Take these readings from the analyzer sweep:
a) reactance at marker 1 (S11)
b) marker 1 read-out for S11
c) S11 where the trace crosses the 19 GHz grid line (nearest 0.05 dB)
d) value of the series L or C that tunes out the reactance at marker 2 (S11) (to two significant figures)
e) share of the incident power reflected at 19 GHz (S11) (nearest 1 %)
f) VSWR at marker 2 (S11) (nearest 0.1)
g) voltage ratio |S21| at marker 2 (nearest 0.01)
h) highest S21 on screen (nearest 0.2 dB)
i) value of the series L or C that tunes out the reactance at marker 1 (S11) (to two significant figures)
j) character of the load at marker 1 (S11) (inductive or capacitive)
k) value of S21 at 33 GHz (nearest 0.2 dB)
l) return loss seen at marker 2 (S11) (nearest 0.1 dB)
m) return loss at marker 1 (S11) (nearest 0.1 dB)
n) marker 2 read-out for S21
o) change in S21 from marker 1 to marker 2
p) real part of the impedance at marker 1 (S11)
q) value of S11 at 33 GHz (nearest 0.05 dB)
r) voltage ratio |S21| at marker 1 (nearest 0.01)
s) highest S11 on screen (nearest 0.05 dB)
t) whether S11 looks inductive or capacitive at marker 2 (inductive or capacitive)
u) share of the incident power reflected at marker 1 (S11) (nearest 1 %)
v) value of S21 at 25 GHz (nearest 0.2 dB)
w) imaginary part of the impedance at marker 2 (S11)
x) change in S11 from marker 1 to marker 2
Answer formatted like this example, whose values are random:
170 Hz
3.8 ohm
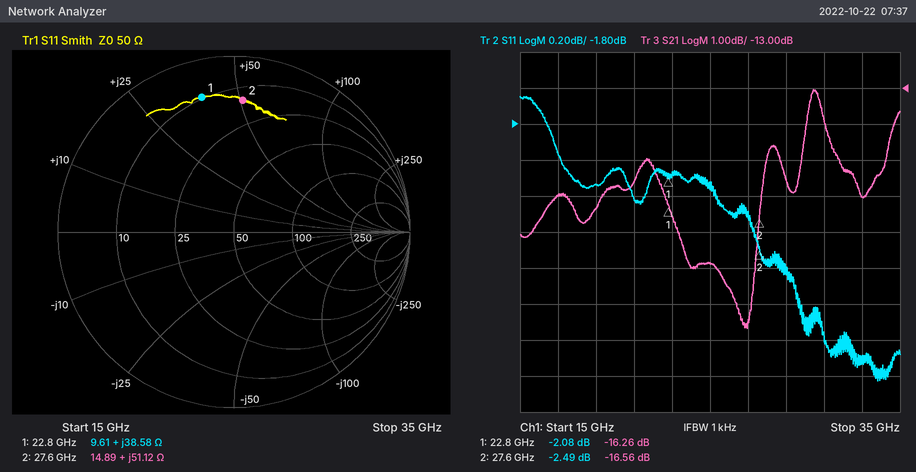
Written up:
+38.58 Ω
-2.08 dB
-2.15 dB
110 fF
61 %
7.0
0.15
-13.0 dB
180 fF
inductive
-16.0 dB
2.5 dB
2.1 dB
-16.56 dB
-0.30 dB
9.61 Ω
-3.10 dB
0.15
-1.65 dB
inductive
62 %
-17.8 dB
+51.12 Ω
-0.41 dB
